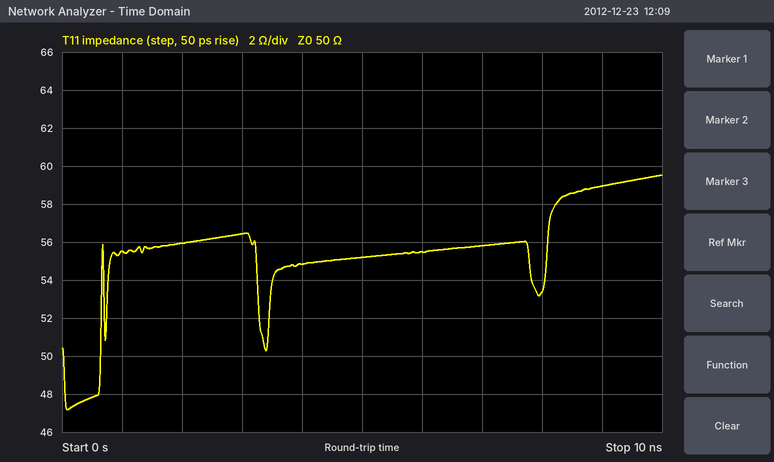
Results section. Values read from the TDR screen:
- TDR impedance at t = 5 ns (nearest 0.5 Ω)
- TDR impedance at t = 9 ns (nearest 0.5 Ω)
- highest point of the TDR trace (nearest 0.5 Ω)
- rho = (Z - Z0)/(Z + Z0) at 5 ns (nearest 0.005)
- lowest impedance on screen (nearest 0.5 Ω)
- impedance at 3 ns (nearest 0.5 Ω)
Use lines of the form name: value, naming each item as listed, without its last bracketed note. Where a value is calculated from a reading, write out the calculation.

TDR impedance at t = 5 ns: 55.0 Ω
TDR impedance at t = 9 ns: 59.0 Ω
highest point of the TDR trace: 59.5 Ω
rho = (Z - Z0)/(Z + Z0) at 5 ns: (55 − 50)/(55 + 50) ≈ +0.0476, so +0.050 to the nearest 0.005
lowest impedance on screen: 47.0 Ω
impedance at 3 ns: 56.5 Ω
